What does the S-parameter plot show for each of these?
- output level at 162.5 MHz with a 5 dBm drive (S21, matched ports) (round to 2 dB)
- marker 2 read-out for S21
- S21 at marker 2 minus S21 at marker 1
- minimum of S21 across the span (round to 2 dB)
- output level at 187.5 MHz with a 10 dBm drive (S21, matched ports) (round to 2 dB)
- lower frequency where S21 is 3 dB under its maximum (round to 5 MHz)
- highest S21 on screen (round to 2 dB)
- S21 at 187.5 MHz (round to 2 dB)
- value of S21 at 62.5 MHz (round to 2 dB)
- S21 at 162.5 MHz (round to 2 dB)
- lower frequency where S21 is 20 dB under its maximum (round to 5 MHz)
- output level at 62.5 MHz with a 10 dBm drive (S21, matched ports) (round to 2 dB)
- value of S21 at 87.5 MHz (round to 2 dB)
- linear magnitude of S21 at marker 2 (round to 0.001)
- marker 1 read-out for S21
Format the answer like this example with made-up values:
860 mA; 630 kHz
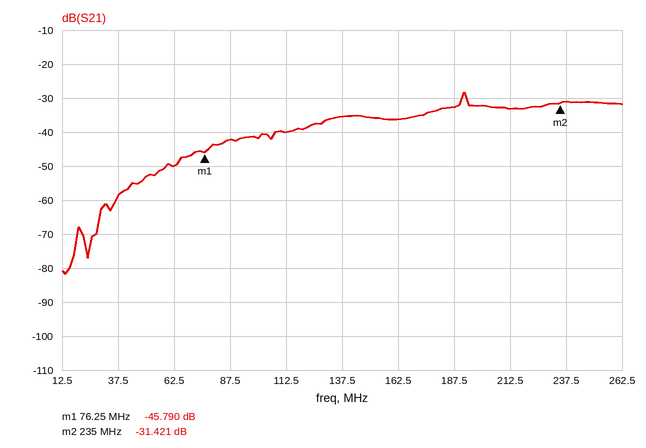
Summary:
-32 dBm; -31.421 dB; 14.369 dB; -82 dB; -22 dBm; 190 MHz; -28 dB; -32 dB; -50 dB; -36 dB; 65 MHz; -40 dBm; -42 dB; 0.027; -45.790 dB
